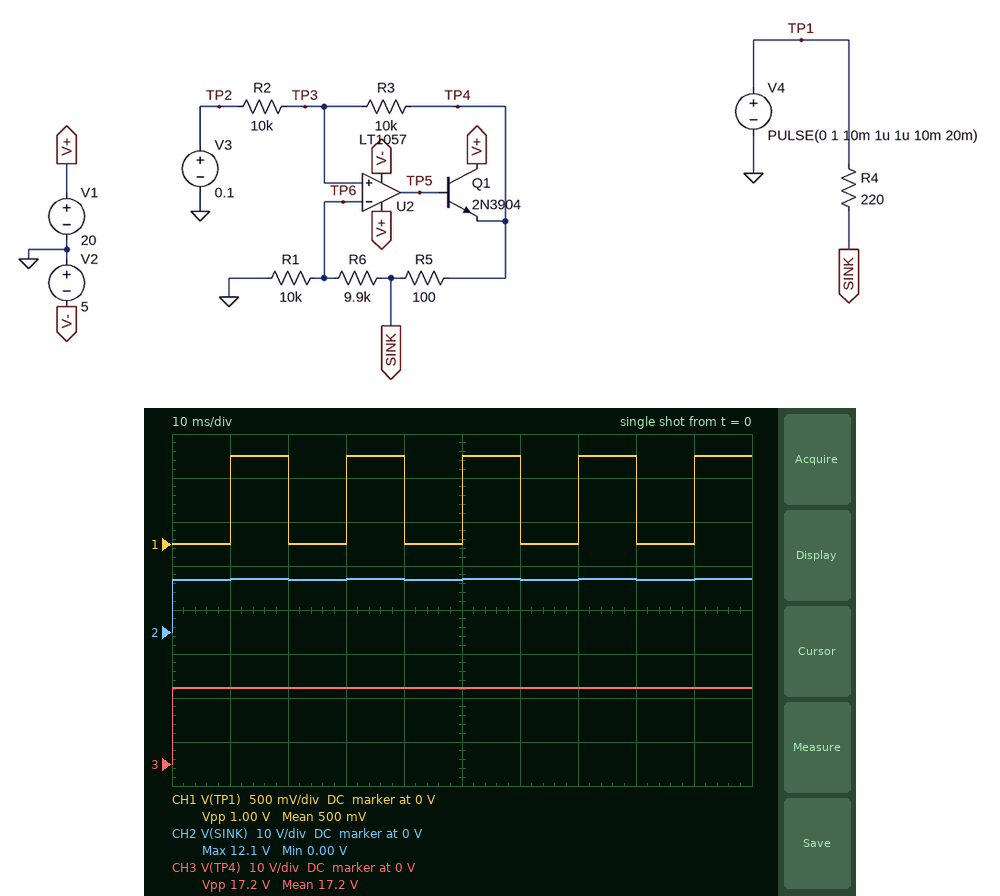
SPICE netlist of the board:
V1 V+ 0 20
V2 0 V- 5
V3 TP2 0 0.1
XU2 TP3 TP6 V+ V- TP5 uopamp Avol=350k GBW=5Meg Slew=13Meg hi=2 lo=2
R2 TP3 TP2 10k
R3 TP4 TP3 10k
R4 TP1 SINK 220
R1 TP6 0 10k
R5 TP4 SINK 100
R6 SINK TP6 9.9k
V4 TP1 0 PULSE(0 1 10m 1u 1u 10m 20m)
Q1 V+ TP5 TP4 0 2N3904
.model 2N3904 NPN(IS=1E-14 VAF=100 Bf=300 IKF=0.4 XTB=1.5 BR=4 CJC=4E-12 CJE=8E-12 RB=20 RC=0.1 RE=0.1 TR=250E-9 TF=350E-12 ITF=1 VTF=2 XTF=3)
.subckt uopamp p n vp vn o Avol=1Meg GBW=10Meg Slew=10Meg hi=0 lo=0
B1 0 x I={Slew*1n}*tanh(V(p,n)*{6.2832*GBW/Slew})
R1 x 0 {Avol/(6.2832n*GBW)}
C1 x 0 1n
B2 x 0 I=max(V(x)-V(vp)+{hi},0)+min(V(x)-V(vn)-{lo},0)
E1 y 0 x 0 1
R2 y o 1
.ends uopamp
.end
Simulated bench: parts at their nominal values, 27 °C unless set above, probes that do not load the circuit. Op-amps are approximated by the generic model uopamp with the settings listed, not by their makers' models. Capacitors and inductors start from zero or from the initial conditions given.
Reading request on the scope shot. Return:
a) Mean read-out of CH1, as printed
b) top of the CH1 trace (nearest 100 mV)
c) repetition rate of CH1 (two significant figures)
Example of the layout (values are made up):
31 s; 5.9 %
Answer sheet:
500 mV; 1.0 V; 50 Hz
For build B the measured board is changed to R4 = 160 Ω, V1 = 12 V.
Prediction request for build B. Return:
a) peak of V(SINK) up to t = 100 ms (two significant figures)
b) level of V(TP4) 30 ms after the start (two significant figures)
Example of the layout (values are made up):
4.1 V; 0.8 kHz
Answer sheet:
6.1 V; 9.3 V
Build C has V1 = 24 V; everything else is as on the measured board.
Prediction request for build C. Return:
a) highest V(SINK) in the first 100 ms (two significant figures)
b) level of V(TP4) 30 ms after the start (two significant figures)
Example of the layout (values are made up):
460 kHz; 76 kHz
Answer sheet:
15 V; 21 V
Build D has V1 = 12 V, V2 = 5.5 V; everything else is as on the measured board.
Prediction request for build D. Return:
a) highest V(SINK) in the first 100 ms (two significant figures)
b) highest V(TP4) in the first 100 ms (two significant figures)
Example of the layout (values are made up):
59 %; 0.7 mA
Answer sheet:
6.7 V; 9.3 V
